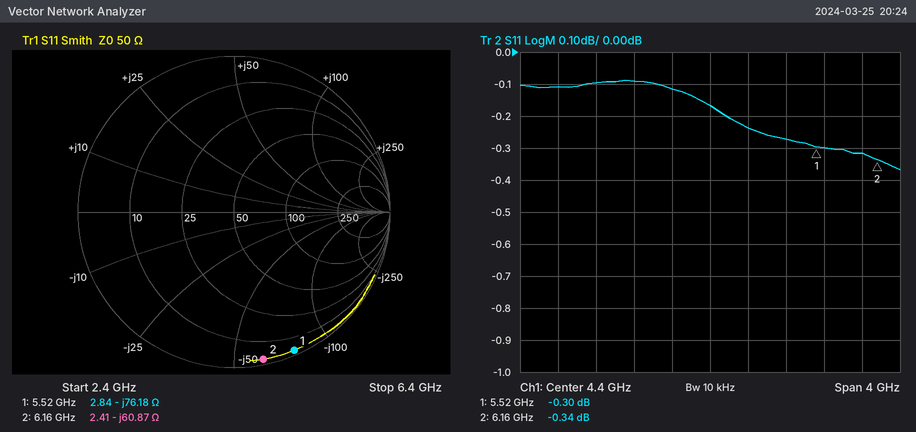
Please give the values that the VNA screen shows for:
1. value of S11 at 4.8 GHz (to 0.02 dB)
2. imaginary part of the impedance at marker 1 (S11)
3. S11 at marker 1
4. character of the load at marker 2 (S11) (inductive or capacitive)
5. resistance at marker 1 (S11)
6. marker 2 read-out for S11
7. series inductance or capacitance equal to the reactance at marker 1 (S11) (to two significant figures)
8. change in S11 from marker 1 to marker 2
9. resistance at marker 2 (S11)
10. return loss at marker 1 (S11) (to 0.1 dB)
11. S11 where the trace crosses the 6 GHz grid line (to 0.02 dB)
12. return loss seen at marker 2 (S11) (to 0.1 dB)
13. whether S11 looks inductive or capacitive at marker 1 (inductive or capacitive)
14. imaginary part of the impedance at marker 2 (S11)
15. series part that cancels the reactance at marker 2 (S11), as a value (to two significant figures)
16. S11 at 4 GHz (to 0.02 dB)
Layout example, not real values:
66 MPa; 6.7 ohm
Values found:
-0.24 dB; -76.18 Ω; -0.30 dB; capacitive; 2.84 Ω; -0.34 dB; 380 fF; -0.04 dB; 2.41 Ω; 0.3 dB; -0.32 dB; 0.3 dB; capacitive; -60.87 Ω; 1.6 nH; -0.12 dB
